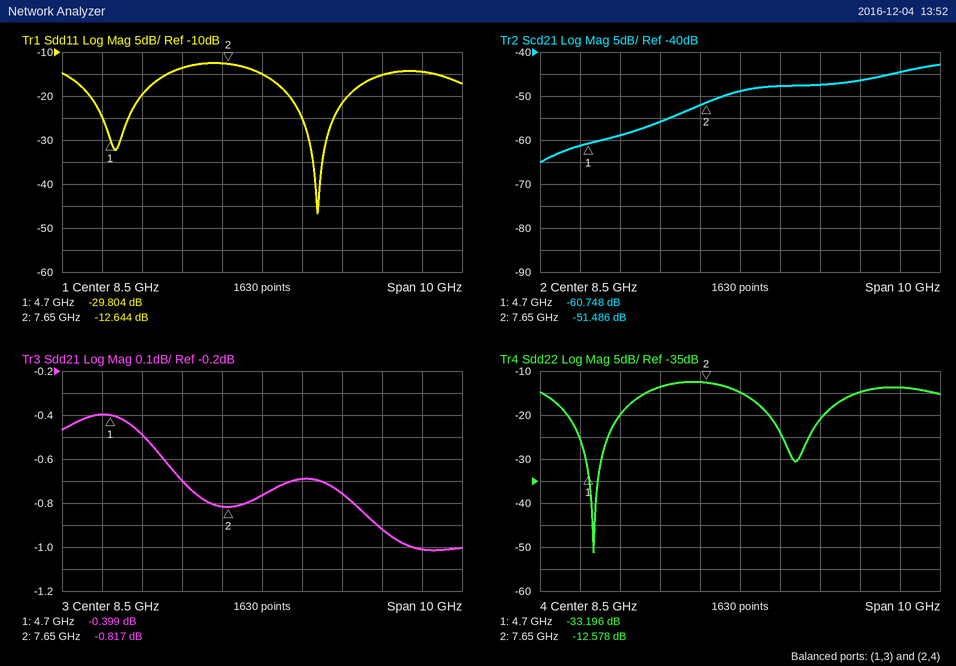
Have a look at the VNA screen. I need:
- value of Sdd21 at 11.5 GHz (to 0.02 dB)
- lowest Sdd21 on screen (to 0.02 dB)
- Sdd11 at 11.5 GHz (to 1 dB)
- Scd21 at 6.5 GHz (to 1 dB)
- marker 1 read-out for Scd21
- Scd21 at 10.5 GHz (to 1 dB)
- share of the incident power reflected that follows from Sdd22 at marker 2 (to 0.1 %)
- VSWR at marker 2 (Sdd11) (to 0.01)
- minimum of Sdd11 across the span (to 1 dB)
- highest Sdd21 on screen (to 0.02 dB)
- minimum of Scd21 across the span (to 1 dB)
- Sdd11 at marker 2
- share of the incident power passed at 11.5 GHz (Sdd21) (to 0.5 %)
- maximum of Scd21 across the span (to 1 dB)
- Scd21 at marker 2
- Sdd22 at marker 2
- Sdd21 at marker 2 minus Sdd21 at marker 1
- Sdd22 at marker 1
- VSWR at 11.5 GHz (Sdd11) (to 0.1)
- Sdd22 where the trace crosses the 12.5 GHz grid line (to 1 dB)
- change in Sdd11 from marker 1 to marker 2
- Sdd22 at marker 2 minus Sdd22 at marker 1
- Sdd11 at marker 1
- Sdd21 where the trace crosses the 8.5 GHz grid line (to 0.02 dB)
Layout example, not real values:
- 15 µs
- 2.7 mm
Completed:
- -0.92 dB
- -1.02 dB
- -15 dB
- -56 dB
- -60.748 dB
- -47 dB
- 5.5 %
- 1.61
- -47 dB
- -0.40 dB
- -65 dB
- -12.644 dB
- 81.0 %
- -43 dB
- -51.486 dB
- -12.578 dB
- -0.418 dB
- -33.196 dB
- 1.4
- -14 dB
- 17.160 dB
- 20.618 dB
- -29.804 dB
- -0.76 dB
